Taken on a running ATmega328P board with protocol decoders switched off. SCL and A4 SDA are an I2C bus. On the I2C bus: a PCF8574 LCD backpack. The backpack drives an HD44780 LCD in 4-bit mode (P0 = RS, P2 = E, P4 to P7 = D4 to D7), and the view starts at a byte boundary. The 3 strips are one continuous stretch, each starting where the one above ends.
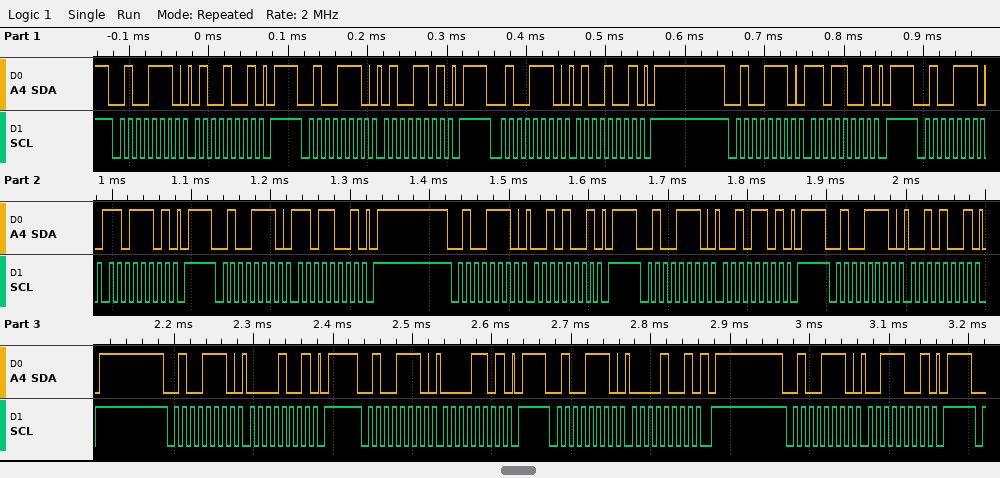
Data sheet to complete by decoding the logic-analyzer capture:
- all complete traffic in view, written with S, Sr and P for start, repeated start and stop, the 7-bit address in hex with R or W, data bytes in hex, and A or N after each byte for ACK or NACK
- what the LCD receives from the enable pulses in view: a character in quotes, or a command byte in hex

S 27W A 49 A P S 27W A 4D A P S 27W A 49 A P S 27W A D9 A P S 27W A DD A P S 27W A D9 A P S 27W A 29 A P S 27W A 2D A P S 27W A 29 A P S 27W A 09 A P S 27W A 0D A P S 27W A 09 A P S 27W A 39 A P
'M' ' '
